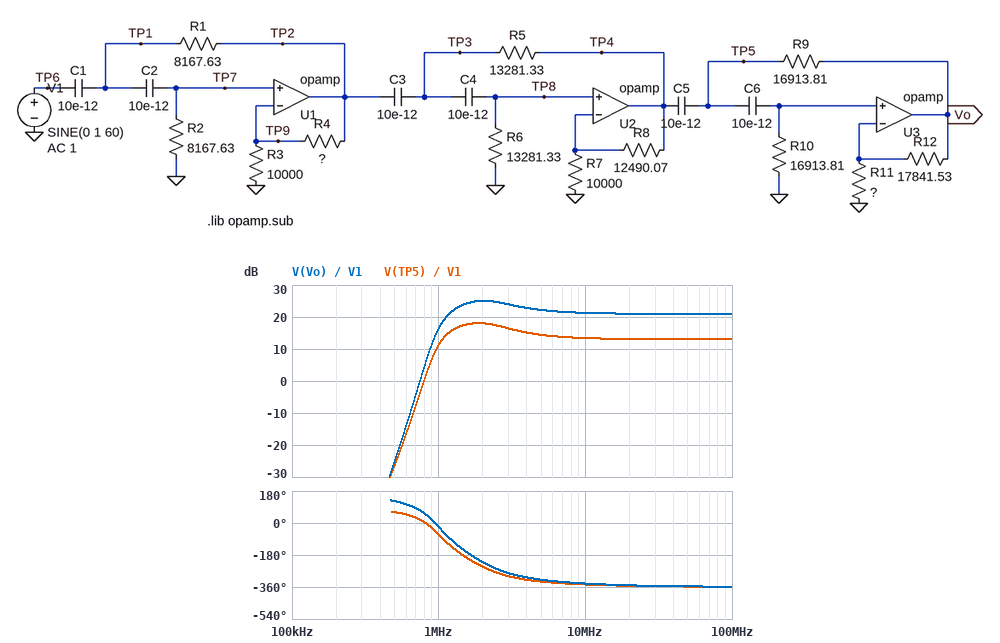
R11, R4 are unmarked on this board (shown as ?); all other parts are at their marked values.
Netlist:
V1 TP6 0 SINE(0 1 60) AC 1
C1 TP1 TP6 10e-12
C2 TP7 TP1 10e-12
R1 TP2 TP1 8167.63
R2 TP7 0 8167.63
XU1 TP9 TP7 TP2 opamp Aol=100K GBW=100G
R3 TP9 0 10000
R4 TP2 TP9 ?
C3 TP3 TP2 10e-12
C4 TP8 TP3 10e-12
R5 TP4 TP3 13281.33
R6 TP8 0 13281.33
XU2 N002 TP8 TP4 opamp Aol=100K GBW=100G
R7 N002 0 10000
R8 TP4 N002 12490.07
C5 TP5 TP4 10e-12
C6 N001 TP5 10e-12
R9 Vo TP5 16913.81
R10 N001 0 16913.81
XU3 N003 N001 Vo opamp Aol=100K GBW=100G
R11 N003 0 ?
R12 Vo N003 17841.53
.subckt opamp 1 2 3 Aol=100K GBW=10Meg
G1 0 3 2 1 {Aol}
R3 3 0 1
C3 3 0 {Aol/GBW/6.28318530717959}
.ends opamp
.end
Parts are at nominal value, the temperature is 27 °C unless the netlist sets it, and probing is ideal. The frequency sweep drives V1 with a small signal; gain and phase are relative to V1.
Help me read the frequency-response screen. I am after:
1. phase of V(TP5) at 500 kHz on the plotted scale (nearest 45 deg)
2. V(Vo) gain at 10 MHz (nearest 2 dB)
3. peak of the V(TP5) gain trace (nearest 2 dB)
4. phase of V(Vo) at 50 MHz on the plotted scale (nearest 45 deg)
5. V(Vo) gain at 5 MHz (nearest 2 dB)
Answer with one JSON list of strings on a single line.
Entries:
["45 deg", "22 dB", "18 dB", "-360 deg", "22 dB"]
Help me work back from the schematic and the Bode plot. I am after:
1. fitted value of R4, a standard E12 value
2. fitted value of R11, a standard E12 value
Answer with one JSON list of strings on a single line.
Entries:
["10 kΩ", "12 kΩ"]
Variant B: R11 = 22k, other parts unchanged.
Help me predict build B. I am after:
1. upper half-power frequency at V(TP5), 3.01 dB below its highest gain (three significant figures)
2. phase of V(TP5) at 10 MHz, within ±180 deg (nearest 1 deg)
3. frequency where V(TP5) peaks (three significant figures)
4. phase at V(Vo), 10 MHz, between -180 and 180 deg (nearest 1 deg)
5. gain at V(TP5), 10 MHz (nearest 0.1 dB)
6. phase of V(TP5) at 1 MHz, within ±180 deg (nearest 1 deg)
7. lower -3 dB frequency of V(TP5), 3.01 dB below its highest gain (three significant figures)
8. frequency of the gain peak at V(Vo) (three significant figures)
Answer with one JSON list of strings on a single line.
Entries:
["6.87 MHz", "18 deg", "2.17 MHz", "23 deg", "13.4 dB", "-58 deg", "1.41 MHz", "2.29 MHz"]
